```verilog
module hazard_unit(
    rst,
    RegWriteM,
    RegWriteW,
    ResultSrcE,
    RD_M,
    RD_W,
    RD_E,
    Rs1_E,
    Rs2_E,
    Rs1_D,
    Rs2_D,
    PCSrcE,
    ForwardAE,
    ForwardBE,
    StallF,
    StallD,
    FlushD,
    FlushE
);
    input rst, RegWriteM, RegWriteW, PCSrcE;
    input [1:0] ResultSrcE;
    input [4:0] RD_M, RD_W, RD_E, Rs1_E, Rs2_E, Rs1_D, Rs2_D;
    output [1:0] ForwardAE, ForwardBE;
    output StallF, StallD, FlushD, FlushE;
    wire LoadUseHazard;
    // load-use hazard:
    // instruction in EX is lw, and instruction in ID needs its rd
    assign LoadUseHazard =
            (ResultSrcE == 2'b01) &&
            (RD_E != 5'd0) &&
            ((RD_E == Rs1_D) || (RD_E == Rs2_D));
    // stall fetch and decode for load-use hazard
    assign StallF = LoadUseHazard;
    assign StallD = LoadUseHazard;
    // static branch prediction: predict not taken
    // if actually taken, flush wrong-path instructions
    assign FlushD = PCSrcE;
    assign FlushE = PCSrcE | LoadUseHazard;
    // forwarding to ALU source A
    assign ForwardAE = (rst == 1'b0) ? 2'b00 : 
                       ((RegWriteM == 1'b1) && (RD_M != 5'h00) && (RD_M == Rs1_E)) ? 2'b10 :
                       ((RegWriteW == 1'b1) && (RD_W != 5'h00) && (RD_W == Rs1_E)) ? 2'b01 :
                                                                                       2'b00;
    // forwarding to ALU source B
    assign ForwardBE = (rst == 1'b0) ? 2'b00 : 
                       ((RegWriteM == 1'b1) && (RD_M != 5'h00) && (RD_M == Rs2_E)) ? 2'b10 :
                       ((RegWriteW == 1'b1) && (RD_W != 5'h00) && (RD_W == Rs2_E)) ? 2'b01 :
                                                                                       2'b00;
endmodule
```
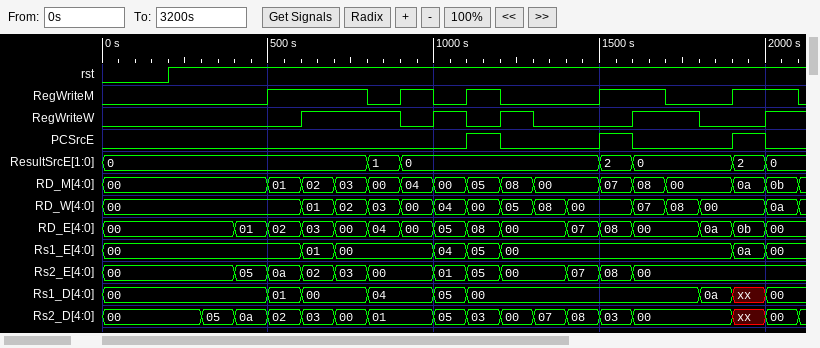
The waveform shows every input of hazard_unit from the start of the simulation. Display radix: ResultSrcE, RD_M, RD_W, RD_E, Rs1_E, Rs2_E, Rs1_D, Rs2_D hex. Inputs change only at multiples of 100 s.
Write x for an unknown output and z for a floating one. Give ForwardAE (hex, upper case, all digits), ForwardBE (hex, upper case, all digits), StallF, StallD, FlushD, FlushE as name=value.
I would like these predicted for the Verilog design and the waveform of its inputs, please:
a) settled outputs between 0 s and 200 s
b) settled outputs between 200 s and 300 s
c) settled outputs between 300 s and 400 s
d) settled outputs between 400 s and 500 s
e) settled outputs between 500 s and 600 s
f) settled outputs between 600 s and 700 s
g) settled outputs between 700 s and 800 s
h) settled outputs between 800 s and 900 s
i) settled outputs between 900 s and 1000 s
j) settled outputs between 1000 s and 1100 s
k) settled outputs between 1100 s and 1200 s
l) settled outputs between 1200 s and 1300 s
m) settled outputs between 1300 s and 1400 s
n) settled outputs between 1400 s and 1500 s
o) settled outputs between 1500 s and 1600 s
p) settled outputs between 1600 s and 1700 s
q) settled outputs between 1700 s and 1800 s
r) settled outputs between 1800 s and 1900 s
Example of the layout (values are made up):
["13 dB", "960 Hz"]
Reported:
["ForwardAE=0, ForwardBE=0, StallF=0, StallD=0, FlushD=0, FlushE=0", "ForwardAE=0, ForwardBE=0, StallF=0, StallD=0, FlushD=0, FlushE=0", "ForwardAE=0, ForwardBE=0, StallF=0, StallD=0, FlushD=0, FlushE=0", "ForwardAE=0, ForwardBE=0, StallF=0, StallD=0, FlushD=0, FlushE=0", "ForwardAE=0, ForwardBE=0, StallF=0, StallD=0, FlushD=0, FlushE=0", "ForwardAE=1, ForwardBE=2, StallF=0, StallD=0, FlushD=0, FlushE=0", "ForwardAE=0, ForwardBE=2, StallF=0, StallD=0, FlushD=0, FlushE=0", "ForwardAE=0, ForwardBE=0, StallF=1, StallD=1, FlushD=0, FlushE=1", "ForwardAE=0, ForwardBE=0, StallF=0, StallD=0, FlushD=0, FlushE=0", "ForwardAE=1, ForwardBE=0, StallF=0, StallD=0, FlushD=0, FlushE=0", "ForwardAE=2, ForwardBE=2, StallF=0, StallD=0, FlushD=1, FlushE=1", "ForwardAE=0, ForwardBE=0, StallF=0, StallD=0, FlushD=0, FlushE=0", "ForwardAE=0, ForwardBE=0, StallF=0, StallD=0, FlushD=0, FlushE=0", "ForwardAE=0, ForwardBE=0, StallF=0, StallD=0, FlushD=0, FlushE=0", "ForwardAE=0, ForwardBE=0, StallF=0, StallD=0, FlushD=1, FlushE=1", "ForwardAE=0, ForwardBE=0, StallF=0, StallD=0, FlushD=0, FlushE=0", "ForwardAE=0, ForwardBE=0, StallF=0, StallD=0, FlushD=0, FlushE=0", "ForwardAE=0, ForwardBE=0, StallF=0, StallD=0, FlushD=0, FlushE=0"]
